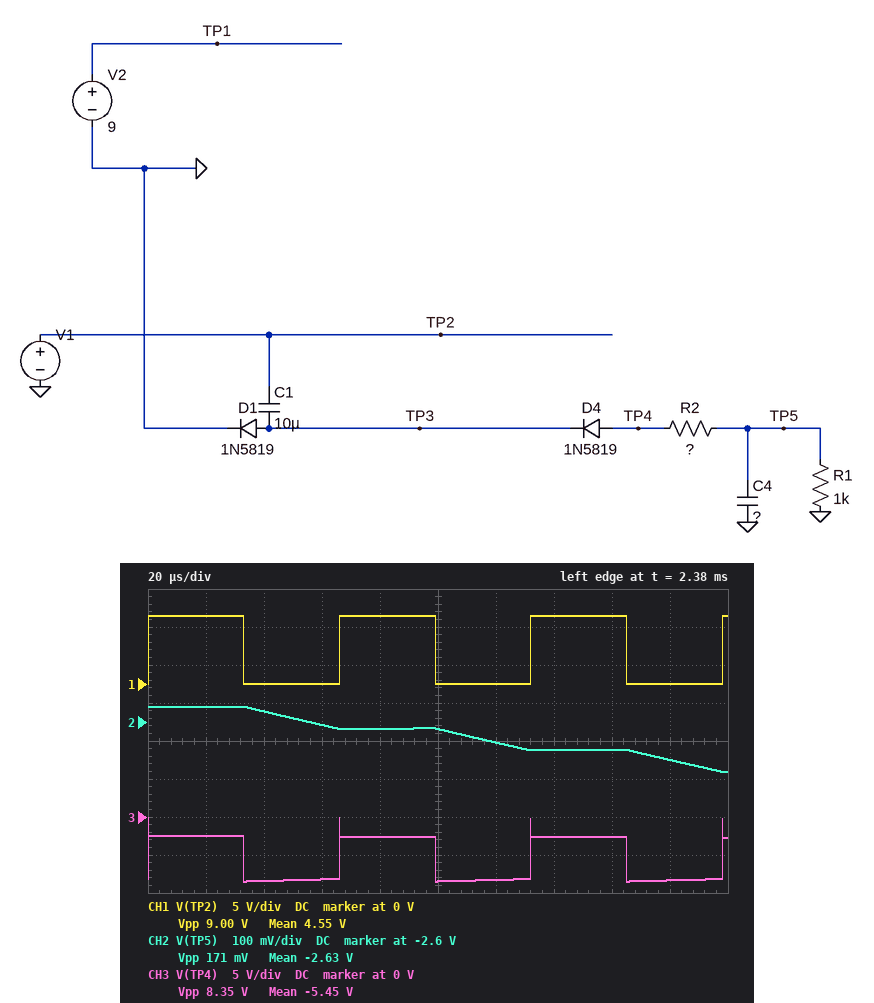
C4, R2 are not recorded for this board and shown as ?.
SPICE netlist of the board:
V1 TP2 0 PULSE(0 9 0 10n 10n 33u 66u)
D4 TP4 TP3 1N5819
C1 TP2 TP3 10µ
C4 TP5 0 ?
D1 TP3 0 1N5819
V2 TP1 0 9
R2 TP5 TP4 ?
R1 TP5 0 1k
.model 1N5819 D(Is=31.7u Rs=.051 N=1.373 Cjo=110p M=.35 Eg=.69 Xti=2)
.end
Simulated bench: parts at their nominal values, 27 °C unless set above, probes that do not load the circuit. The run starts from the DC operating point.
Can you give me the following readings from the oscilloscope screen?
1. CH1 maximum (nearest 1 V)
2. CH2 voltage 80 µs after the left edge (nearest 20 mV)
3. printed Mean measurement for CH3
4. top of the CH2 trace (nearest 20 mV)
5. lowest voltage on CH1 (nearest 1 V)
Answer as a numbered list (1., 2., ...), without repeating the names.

1. 9 V
2. -2.62 V
3. -5.45 V
4. -2.56 V
5. 0 V
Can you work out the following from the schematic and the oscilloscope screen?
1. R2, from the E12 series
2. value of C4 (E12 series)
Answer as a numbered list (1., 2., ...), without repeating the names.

1. 56 Ω
2. 56 µF
